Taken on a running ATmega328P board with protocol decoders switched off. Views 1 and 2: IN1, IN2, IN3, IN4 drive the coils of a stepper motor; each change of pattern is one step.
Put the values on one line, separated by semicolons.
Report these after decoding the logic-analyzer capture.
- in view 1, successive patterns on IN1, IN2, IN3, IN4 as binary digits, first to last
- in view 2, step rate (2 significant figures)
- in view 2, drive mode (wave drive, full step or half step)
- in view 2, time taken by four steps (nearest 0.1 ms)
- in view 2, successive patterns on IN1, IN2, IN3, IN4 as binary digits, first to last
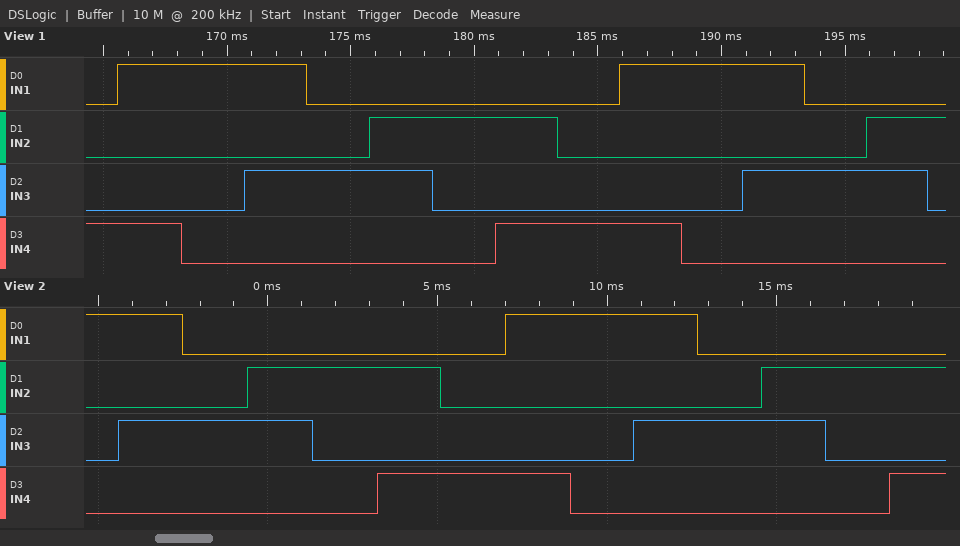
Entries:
0001 1001 1000 1010 0010 0110 0100 0101 0001 1001 1000 1010 0010 0110 0100; 530 steps/s; half step; 7.6 ms; 1000 1010 0010 0110 0100 0101 0001 1001 1000 1010 0010 0110 0100 0101
